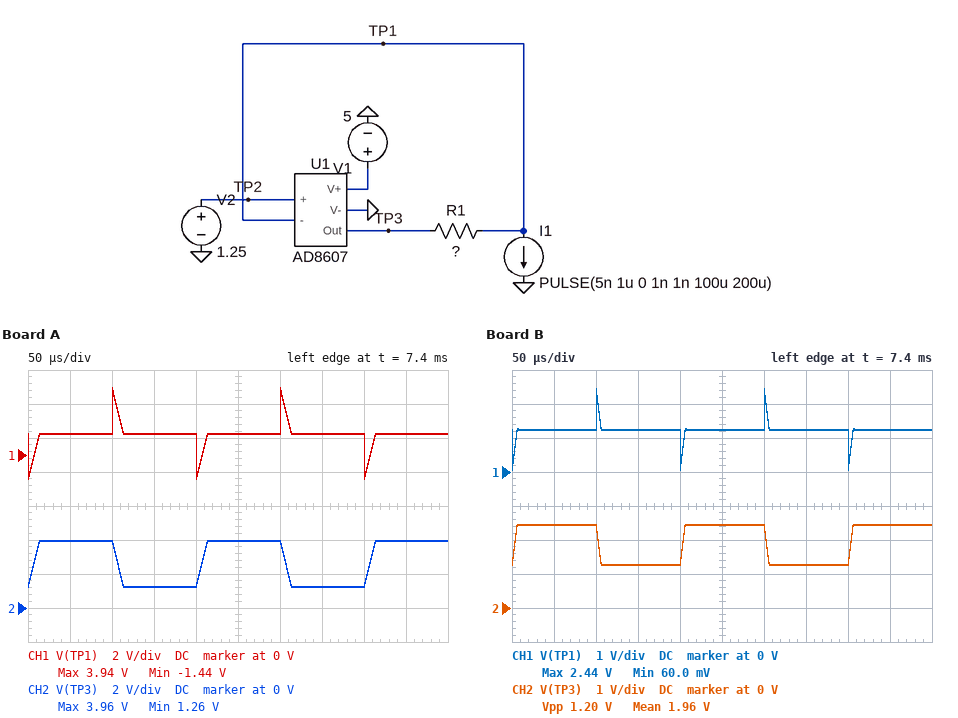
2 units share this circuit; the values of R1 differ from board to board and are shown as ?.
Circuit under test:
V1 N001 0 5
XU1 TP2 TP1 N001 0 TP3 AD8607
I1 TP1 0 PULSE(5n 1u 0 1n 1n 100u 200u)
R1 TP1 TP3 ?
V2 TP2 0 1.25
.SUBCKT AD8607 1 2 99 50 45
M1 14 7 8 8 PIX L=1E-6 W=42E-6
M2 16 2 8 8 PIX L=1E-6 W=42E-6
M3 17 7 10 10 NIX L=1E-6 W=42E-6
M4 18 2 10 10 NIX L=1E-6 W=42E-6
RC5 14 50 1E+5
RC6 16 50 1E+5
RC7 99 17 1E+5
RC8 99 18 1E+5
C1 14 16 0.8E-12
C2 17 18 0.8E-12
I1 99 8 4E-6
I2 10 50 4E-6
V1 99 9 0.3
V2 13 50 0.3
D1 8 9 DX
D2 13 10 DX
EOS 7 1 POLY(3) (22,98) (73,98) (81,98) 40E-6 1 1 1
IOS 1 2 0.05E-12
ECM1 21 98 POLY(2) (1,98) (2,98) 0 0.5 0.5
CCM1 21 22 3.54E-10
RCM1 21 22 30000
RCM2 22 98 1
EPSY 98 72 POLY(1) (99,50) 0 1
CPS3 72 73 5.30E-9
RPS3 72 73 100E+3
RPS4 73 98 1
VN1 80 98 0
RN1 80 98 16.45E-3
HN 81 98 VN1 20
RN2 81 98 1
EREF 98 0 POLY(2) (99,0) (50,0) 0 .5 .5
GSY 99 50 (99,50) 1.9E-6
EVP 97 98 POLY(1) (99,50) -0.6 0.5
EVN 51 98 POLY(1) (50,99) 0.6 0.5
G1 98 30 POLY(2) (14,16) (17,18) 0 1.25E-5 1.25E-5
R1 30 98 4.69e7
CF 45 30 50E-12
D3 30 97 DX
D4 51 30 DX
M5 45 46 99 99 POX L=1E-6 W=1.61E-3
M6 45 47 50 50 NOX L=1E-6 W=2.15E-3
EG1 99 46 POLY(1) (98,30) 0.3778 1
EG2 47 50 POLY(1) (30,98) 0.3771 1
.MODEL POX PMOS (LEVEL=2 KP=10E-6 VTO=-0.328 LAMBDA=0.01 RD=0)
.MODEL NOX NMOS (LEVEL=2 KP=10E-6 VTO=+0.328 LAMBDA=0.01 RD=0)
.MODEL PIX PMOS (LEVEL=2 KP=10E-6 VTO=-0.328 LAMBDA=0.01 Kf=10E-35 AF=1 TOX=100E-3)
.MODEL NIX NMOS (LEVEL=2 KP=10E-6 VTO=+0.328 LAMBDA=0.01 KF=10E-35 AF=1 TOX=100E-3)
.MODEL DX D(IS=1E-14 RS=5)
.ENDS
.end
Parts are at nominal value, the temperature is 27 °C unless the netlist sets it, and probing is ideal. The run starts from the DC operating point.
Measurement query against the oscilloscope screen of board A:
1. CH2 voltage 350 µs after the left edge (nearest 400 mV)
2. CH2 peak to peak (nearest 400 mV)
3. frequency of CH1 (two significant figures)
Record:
1.2 V
2.8 V
5.0 kHz
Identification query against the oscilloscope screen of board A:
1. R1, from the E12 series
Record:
2.7 MΩ
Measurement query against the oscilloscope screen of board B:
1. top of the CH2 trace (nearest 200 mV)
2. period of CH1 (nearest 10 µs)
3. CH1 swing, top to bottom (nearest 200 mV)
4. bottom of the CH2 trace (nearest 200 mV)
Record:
2.4 V
200 µs
2.4 V
1.2 V
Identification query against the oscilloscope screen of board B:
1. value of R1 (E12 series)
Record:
1.2 MΩ
